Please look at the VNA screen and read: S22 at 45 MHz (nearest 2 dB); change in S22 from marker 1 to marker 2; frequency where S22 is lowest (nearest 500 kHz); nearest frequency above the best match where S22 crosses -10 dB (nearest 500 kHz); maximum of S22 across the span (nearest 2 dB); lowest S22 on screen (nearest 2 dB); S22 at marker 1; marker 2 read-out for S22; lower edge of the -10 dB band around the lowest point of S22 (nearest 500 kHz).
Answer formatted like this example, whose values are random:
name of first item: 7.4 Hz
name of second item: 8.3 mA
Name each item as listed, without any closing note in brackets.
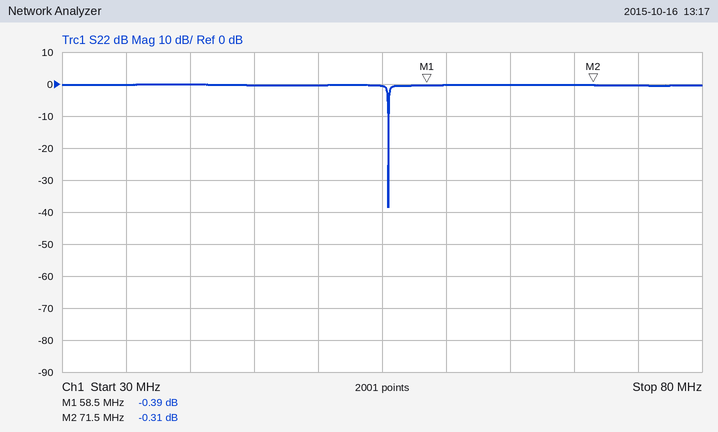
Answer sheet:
S22 at 45 MHz: 0 dB
change in S22 from marker 1 to marker 2: 0.08 dB
frequency where S22 is lowest: 55.5 MHz
nearest frequency above the best match where S22 crosses -10 dB: 55.5 MHz
maximum of S22 across the span: 0 dB
lowest S22 on screen: -38 dB
S22 at marker 1: -0.39 dB
marker 2 read-out for S22: -0.31 dB
lower edge of the -10 dB band around the lowest point of S22: 55.5 MHz
